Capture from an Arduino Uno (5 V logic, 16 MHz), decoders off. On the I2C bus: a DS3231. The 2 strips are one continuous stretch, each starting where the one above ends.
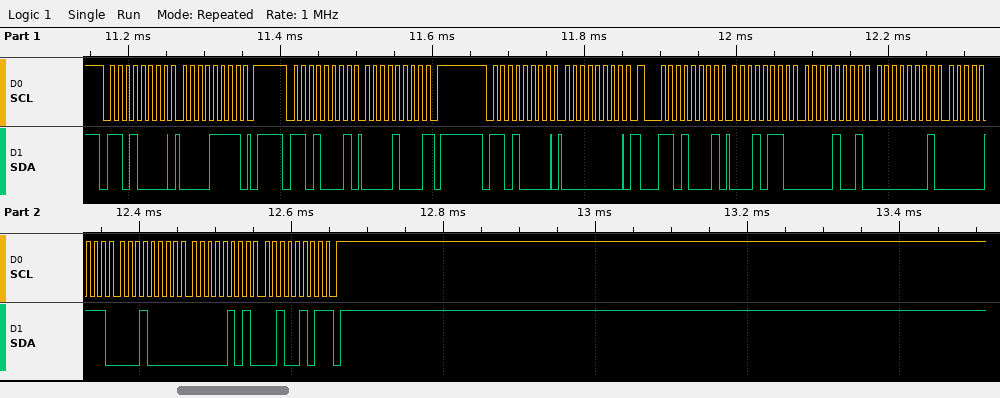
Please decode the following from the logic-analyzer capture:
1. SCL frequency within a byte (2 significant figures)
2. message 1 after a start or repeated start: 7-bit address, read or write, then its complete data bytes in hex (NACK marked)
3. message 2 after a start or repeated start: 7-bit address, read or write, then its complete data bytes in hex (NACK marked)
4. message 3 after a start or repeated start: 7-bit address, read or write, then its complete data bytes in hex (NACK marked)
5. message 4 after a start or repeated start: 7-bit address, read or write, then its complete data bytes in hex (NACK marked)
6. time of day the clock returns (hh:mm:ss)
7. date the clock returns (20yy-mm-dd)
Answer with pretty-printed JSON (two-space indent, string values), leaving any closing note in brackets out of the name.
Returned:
{
  "SCL frequency within a byte": "100 kHz",
  "message 1 after a start or repeated start: 7-bit address, read or write, then its complete data bytes in hex": "0x68 write: 0F",
  "message 2 after a start or repeated start: 7-bit address, read or write, then its complete data bytes in hex": "0x68 read: 08 NACK",
  "message 3 after a start or repeated start: 7-bit address, read or write, then its complete data bytes in hex": "0x68 write: 00",
  "message 4 after a start or repeated start: 7-bit address, read or write, then its complete data bytes in hex": "0x68 read: 16 09 01 07 10 05 25 NACK",
  "time of day the clock returns": "01:09:16",
  "date the clock returns": "2025-05-10"
}
